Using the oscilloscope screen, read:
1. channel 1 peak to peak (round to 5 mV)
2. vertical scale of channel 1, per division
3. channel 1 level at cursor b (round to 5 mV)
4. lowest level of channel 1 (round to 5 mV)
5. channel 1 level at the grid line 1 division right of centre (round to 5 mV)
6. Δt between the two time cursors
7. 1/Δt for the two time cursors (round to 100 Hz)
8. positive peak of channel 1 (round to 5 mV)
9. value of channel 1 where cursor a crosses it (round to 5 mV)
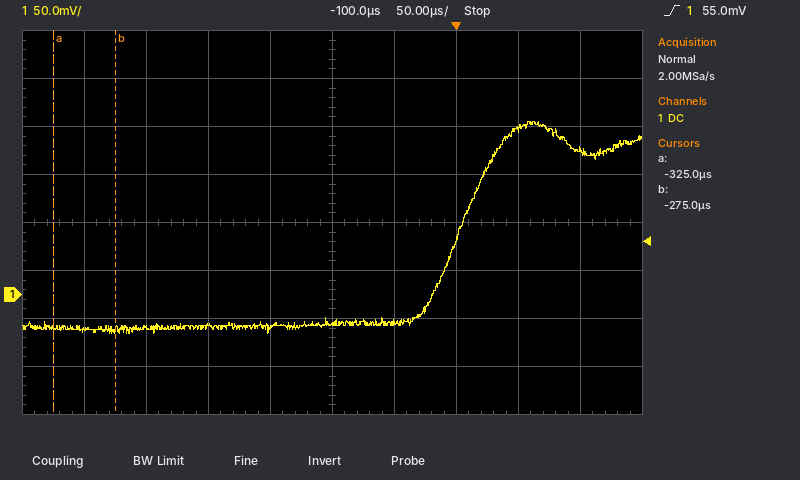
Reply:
220 mV
50 mV
-35 mV
-40 mV
-30 mV
50 µs
20.0 kHz
180 mV
-35 mV
